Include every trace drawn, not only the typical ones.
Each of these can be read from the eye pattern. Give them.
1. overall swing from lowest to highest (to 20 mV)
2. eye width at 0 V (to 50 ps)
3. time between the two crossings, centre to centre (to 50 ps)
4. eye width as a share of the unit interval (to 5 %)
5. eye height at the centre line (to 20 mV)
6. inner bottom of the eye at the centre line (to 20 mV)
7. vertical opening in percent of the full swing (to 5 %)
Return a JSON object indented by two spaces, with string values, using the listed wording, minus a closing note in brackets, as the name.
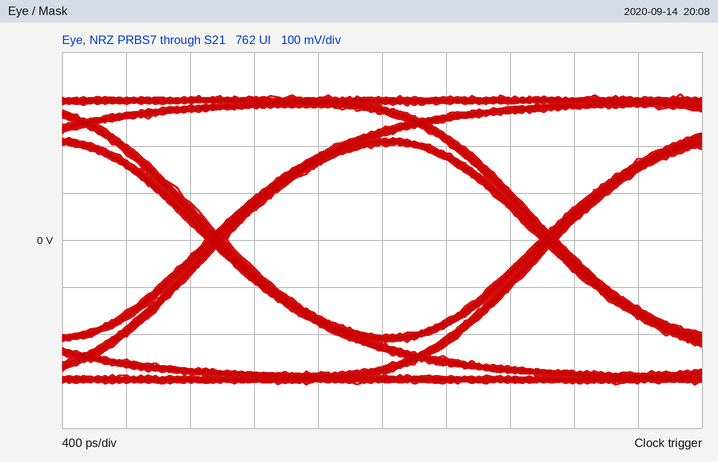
{
  "overall swing from lowest to highest": "620 mV",
  "eye width at 0 V": "1.95 ns",
  "time between the two crossings, centre to centre": "2.10 ns",
  "eye width as a share of the unit interval": "95 %",
  "eye height at the centre line": "400 mV",
  "inner bottom of the eye at the centre line": "-200 mV",
  "vertical opening in percent of the full swing": "65 %"
}
